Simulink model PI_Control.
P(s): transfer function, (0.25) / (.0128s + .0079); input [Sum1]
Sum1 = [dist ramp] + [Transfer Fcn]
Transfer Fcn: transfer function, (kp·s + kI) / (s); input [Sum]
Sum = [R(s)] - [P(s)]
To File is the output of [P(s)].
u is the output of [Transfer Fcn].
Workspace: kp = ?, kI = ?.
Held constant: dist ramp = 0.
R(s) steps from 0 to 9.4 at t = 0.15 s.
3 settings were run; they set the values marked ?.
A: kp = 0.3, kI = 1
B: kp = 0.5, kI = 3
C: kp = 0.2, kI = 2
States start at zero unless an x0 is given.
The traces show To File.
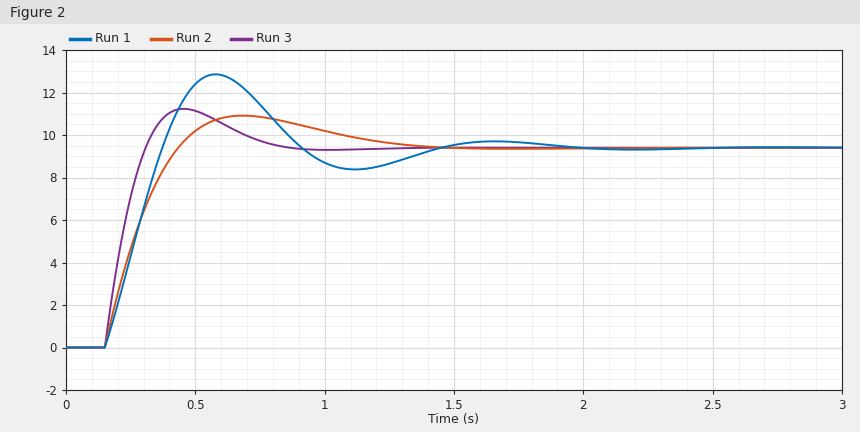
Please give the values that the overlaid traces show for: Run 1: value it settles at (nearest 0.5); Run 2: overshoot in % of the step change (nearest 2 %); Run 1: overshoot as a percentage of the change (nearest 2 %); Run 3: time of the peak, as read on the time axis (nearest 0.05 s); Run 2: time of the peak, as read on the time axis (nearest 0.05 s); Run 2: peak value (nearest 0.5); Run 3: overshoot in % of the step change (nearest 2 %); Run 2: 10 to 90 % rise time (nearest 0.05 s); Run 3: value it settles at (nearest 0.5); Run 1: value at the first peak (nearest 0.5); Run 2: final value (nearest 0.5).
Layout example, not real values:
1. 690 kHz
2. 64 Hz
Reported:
1. 9.5
2. 16 %
3. 36 %
4. 0.45 s
5. 0.70 s
6. 11.0
7. 20 %
8. 0.20 s
9. 9.5
10. 13.0
11. 9.5
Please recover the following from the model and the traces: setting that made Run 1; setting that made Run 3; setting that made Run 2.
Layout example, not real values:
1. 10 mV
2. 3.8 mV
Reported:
1. C
2. B
3. A
